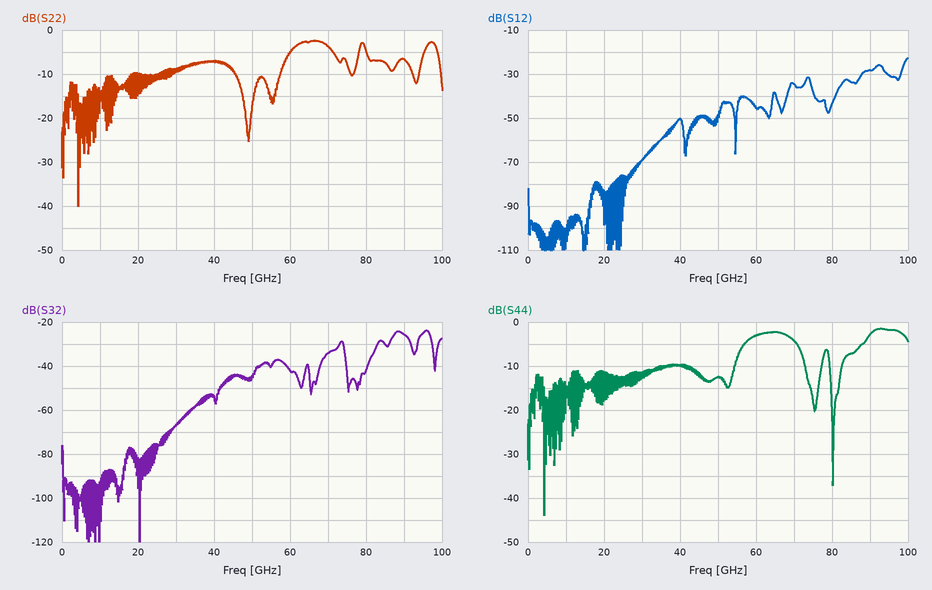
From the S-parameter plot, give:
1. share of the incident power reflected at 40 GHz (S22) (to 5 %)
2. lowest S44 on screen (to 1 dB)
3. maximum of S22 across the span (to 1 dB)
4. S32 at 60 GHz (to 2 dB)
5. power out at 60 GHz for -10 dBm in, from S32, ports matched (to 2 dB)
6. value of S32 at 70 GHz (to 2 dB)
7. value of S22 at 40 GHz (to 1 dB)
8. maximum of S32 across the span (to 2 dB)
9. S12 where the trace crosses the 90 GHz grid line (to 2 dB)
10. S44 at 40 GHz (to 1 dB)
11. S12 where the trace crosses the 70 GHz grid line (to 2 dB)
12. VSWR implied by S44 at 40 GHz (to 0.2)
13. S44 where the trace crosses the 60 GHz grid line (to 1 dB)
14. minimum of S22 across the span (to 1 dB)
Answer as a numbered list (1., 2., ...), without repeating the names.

1. 20 %
2. -44 dB
3. -2 dB
4. -42 dB
5. -52 dBm
6. -34 dB
7. -7 dB
8. -24 dB
9. -28 dB
10. -10 dB
11. -34 dB
12. 2.0
13. -3 dB
14. -40 dB
